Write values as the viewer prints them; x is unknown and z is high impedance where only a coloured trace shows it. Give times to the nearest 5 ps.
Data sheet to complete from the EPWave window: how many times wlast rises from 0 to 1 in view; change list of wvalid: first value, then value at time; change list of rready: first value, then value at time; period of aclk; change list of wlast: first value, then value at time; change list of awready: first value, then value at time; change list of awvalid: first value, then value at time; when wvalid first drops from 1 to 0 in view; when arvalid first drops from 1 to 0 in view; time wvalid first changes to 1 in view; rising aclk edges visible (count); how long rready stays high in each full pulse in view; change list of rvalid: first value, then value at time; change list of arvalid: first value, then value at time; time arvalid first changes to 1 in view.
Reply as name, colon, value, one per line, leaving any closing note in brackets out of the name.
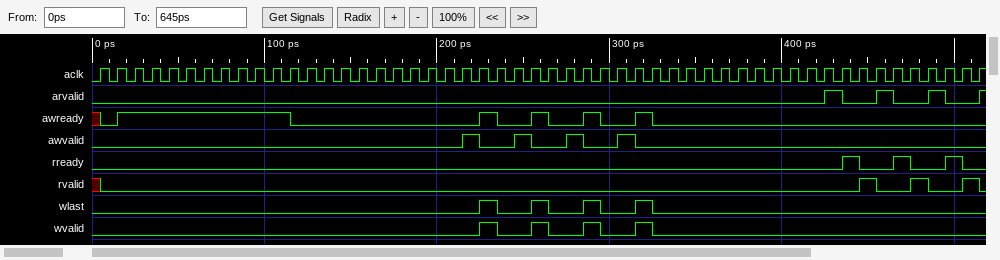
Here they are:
how many times wlast rises from 0 to 1 in view: 4
change list of wvalid: first value, then value at time: 0, 1 at 225 ps, 0 at 235 ps, 1 at 255 ps, 0 at 265 ps, 1 at 285 ps, 0 at 295 ps, 1 at 315 ps, 0 at 325 ps
change list of rready: first value, then value at time: 0, 1 at 435 ps, 0 at 445 ps, 1 at 465 ps, 0 at 475 ps, 1 at 495 ps, 0 at 505 ps
period of aclk: 10 ps
change list of wlast: first value, then value at time: 0, 1 at 225 ps, 0 at 235 ps, 1 at 255 ps, 0 at 265 ps, 1 at 285 ps, 0 at 295 ps, 1 at 315 ps, 0 at 325 ps
change list of awready: first value, then value at time: x, 0 at 5 ps, 1 at 15 ps, 0 at 115 ps, 1 at 225 ps, 0 at 235 ps, 1 at 255 ps, 0 at 265 ps, 1 at 285 ps, 0 at 295 ps, 1 at 315 ps, 0 at 325 ps
change list of awvalid: first value, then value at time: 0, 1 at 215 ps, 0 at 225 ps, 1 at 245 ps, 0 at 255 ps, 1 at 275 ps, 0 at 285 ps, 1 at 305 ps, 0 at 315 ps
when wvalid first drops from 1 to 0 in view: 235 ps
when arvalid first drops from 1 to 0 in view: 435 ps
time wvalid first changes to 1 in view: 225 ps
rising aclk edges visible: 52
how long rready stays high in each full pulse in view: 10 ps, 10 ps, 10 ps
change list of rvalid: first value, then value at time: x, 0 at 5 ps, 1 at 445 ps, 0 at 455 ps, 1 at 475 ps, 0 at 485 ps, 1 at 505 ps, 0 at 515 ps
change list of arvalid: first value, then value at time: 0, 1 at 425 ps, 0 at 435 ps, 1 at 455 ps, 0 at 465 ps, 1 at 485 ps, 0 at 495 ps, 1 at 515 ps
time arvalid first changes to 1 in view: 425 ps
